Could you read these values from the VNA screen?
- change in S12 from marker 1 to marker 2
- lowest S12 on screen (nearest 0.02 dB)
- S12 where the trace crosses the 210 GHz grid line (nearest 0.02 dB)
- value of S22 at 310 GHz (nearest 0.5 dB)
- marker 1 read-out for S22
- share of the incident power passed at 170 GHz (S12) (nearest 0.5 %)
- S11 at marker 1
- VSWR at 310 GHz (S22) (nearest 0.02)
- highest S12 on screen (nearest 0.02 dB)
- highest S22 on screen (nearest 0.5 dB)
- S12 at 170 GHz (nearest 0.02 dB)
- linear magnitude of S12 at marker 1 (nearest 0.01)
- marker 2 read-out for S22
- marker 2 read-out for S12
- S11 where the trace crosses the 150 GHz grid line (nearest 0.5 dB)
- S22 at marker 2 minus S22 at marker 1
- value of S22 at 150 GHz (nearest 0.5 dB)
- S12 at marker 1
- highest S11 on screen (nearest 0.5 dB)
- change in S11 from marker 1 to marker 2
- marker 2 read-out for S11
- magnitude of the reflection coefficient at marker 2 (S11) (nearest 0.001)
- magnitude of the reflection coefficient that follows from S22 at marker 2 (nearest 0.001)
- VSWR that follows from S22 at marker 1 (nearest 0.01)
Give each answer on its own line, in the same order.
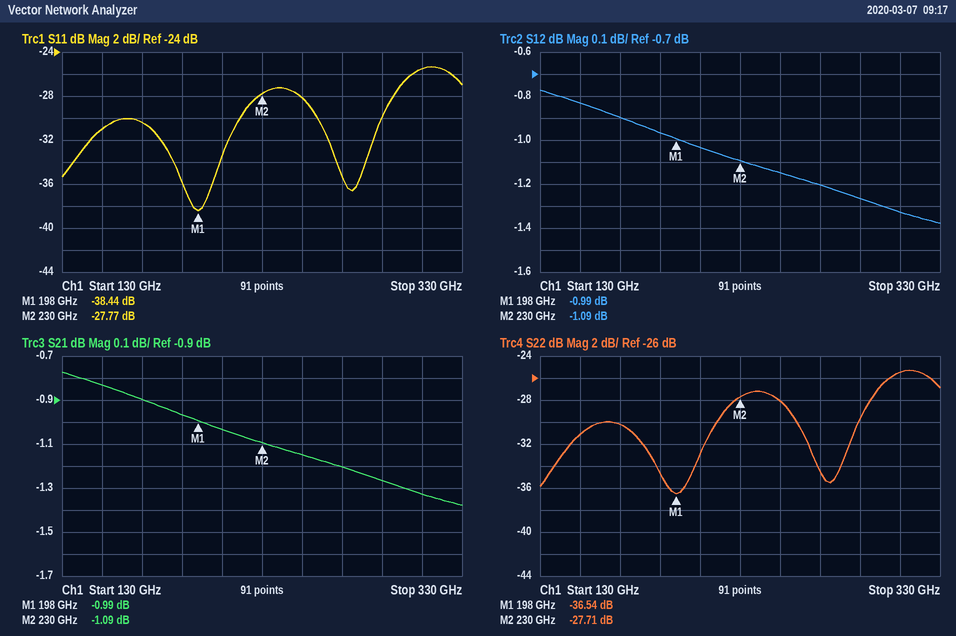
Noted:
-0.10 dB
-1.38 dB
-1.04 dB
-25.5 dB
-36.54 dB
81.5 %
-38.44 dB
1.12
-0.78 dB
-25.5 dB
-0.90 dB
0.89
-27.71 dB
-1.09 dB
-31.0 dB
8.83 dB
-31.0 dB
-0.99 dB
-25.5 dB
10.67 dB
-27.77 dB
0.041
0.041
1.03
